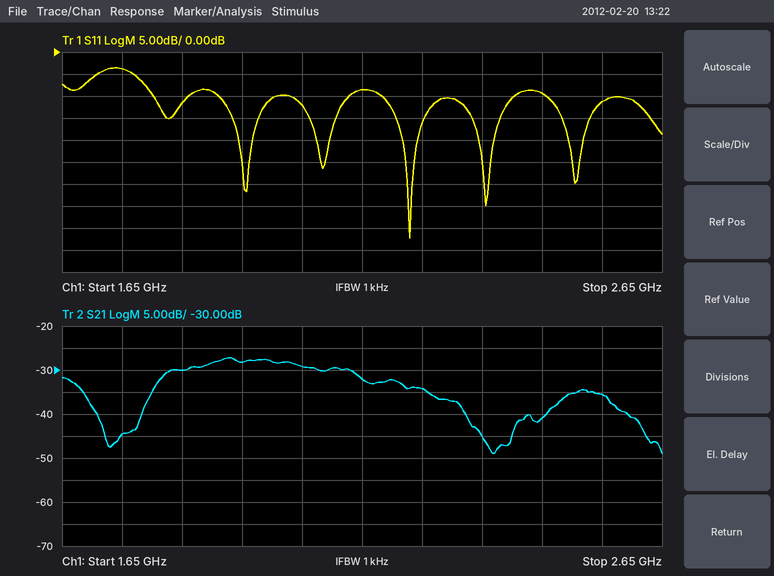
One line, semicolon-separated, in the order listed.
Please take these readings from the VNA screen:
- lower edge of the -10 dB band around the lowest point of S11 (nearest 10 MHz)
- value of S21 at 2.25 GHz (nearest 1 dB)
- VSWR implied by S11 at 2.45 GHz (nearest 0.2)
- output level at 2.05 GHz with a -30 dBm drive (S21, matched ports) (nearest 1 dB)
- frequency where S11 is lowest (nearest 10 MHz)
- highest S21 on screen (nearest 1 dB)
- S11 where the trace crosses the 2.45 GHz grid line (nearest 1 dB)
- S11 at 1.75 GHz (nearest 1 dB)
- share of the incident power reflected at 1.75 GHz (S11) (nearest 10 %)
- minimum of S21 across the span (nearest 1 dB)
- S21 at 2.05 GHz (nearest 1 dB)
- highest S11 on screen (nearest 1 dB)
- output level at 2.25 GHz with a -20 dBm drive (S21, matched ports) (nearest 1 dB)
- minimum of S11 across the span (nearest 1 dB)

2.18 GHz; -34 dB; 2.0; -59 dBm; 2.23 GHz; -27 dB; -9 dB; -4 dB; 40 %; -49 dB; -29 dB; -4 dB; -54 dBm; -42 dB
